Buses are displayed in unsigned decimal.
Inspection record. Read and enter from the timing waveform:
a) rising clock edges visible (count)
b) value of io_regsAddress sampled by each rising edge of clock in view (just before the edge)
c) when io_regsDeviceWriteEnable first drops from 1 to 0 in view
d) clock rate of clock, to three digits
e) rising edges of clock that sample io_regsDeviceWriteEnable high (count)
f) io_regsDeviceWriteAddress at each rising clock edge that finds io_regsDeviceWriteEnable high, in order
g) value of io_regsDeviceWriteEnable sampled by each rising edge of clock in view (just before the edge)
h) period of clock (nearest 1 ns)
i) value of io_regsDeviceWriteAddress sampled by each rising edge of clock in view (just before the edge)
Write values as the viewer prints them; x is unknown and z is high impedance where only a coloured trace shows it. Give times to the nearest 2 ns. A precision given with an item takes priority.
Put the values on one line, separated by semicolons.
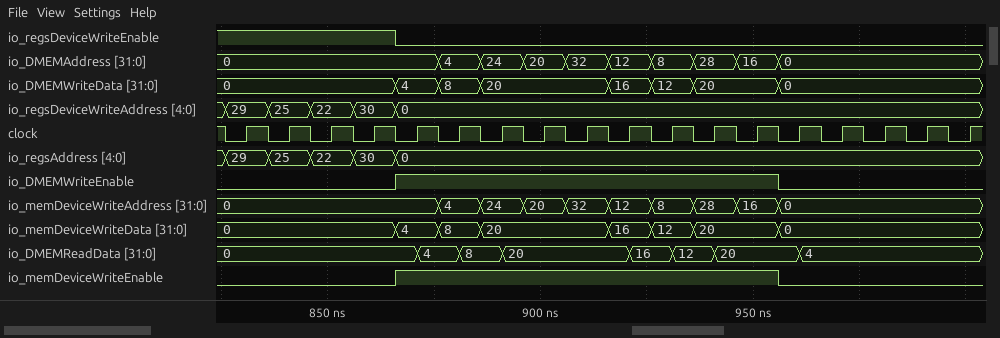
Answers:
18; 29, 25, 22, 30, 0, 0, 0, 0, 0, 0, 0, 0, 0, 0, 0, 0, 0, 0; 866 ns; 100 MHz; 4; 29, 25, 22, 30; 1 1 1 1 0 0 0 0 0 0 0 0 0 0 0 0 0 0; 10 ns; 29, 25, 22, 30, 0, 0, 0, 0, 0, 0, 0, 0, 0, 0, 0, 0, 0, 0
